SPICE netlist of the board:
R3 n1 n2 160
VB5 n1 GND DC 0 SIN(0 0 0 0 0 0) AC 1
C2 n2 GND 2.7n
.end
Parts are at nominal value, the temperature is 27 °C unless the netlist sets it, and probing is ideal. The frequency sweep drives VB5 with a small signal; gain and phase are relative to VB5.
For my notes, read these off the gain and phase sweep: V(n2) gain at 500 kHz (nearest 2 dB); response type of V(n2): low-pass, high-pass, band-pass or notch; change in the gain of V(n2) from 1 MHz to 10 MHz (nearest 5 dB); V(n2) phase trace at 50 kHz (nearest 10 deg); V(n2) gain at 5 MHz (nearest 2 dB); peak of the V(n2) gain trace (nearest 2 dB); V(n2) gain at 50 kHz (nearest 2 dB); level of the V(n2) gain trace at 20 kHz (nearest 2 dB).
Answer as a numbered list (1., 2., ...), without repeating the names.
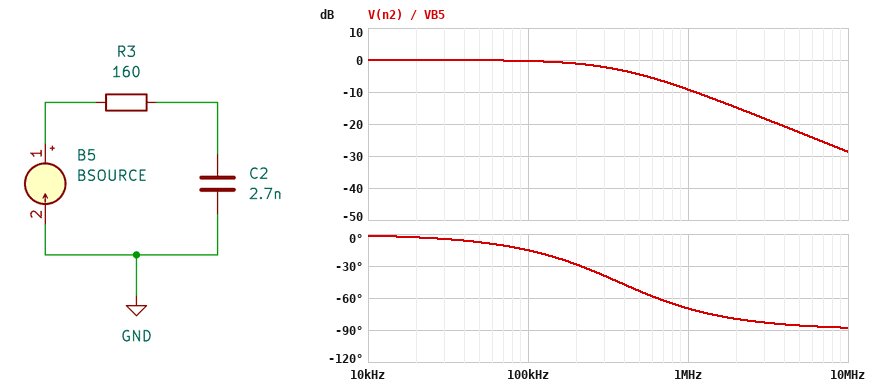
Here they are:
1. -4 dB
2. low-pass
3. -20 dB
4. -10 deg
5. -22 dB
6. 0 dB
7. 0 dB
8. 0 dB
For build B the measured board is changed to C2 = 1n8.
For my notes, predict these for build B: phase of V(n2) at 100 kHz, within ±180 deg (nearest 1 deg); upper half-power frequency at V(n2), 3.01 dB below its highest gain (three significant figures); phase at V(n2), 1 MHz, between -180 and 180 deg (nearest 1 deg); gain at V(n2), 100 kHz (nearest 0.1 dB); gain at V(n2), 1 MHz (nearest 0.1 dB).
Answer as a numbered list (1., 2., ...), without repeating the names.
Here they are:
1. -10 deg
2. 553 kHz
3. -61 deg
4. -0.1 dB
5. -6.3 dB
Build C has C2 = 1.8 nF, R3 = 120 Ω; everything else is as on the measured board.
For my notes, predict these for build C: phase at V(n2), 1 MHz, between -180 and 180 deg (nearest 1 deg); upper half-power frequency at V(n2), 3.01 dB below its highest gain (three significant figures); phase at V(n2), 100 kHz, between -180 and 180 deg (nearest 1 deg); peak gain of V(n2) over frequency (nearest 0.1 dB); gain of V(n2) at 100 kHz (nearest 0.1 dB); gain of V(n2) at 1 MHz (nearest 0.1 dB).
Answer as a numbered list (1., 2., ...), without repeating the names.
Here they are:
1. -54 deg
2. 737 kHz
3. -8 deg
4. 0 dB
5. -0.1 dB
6. -4.5 dB
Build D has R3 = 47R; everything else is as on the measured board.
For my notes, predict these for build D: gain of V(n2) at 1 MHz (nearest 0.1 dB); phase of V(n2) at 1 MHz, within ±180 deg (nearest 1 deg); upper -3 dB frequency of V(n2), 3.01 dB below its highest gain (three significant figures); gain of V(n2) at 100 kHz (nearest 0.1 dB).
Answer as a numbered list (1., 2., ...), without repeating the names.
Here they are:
1. -2.1 dB
2. -39 deg
3. 1.25 MHz
4. 0 dB
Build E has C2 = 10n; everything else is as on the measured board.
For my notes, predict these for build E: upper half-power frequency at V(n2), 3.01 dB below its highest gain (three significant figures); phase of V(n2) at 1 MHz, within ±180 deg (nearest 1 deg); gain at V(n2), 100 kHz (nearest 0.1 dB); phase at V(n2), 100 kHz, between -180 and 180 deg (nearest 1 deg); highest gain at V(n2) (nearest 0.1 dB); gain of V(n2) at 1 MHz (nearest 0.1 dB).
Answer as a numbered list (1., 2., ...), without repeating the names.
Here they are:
1. 99.5 kHz
2. -84 deg
3. -3.0 dB
4. -45 deg
5. 0 dB
6. -20.1 dB
